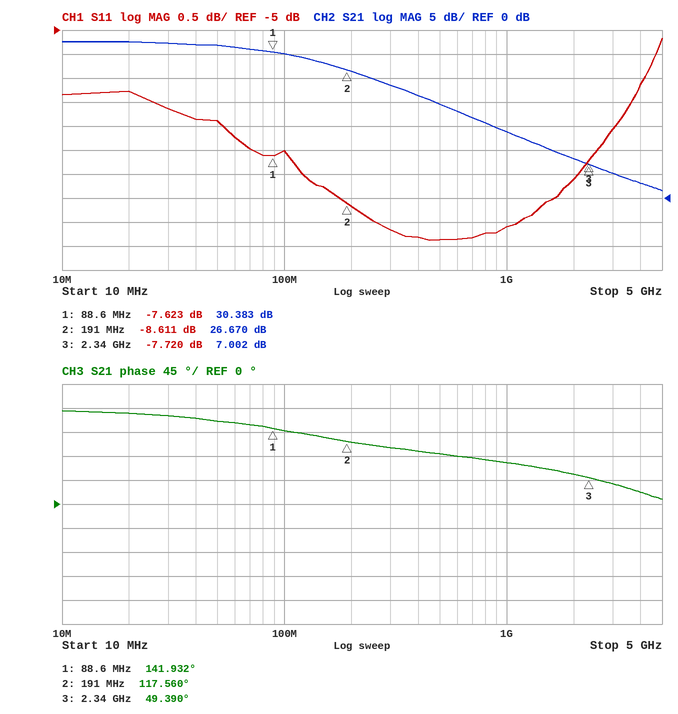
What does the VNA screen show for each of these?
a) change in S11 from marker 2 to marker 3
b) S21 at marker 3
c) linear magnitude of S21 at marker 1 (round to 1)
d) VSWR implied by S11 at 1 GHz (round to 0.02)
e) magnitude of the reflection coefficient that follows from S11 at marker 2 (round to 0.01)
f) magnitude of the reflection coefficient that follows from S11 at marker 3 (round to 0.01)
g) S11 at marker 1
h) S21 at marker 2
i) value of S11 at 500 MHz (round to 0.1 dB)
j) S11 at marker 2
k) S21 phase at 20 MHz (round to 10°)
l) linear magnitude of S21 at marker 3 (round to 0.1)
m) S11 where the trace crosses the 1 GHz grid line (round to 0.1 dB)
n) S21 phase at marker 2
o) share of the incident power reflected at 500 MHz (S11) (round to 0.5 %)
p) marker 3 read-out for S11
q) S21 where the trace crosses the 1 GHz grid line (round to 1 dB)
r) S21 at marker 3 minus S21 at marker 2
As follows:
0.891 dB
7.002 dB
33
2.08
0.37
0.41
-7.623 dB
26.670 dB
-9.4 dB
-8.611 dB
170°
2.2
-9.1 dB
117.560°
11.5 %
-7.720 dB
14 dB
-19.668 dB
